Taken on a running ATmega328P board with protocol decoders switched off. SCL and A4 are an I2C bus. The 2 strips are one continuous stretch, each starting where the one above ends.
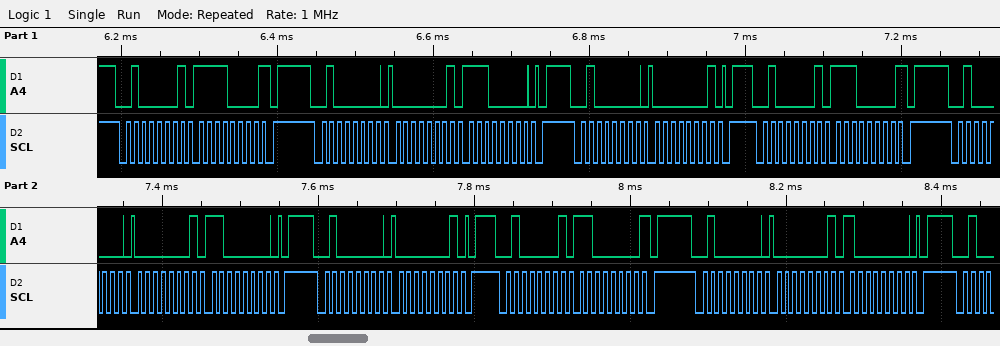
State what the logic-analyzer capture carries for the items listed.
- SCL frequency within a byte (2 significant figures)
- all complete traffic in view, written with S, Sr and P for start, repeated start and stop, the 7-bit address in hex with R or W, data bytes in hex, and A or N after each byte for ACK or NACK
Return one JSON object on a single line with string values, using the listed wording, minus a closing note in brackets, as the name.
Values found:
{"SCL frequency within a byte": "100 kHz", "all complete traffic in view, written with S, Sr and P for start, repeated start and stop, the 7-bit address in hex with R or W, data bytes in hex, and A or N after each byte for ACK or NACK": "S 20R A F0 N P S 20W A 01 A E0 A P S 20W A 01 A P S 20R A E0 N P S 20W A 01 A C0 A P S 20W A 01 A P S 20R A C0 N P S 20W A 01 A 80 A P"}
